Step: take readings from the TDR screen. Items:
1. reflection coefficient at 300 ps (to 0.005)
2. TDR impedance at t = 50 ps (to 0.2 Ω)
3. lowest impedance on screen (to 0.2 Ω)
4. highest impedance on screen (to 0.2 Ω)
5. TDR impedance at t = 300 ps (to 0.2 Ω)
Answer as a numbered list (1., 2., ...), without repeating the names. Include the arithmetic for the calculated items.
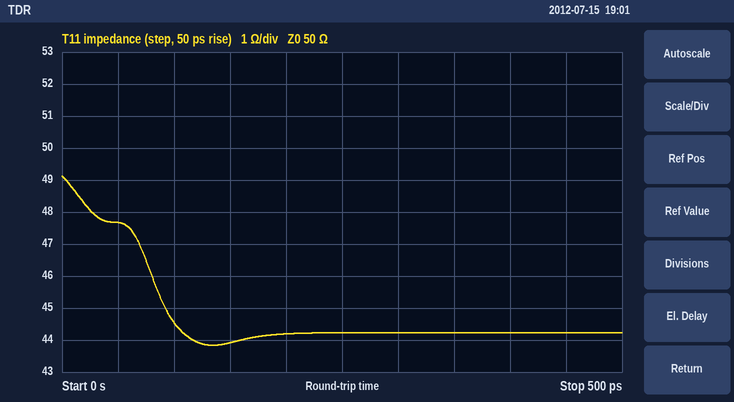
1. (44.2 − 50)/(44.2 + 50) ≈ -0.0616, so -0.060 to the nearest 0.005
2. 47.6 Ω
3. 43.8 Ω
4. 49.2 Ω
5. 44.2 Ω
